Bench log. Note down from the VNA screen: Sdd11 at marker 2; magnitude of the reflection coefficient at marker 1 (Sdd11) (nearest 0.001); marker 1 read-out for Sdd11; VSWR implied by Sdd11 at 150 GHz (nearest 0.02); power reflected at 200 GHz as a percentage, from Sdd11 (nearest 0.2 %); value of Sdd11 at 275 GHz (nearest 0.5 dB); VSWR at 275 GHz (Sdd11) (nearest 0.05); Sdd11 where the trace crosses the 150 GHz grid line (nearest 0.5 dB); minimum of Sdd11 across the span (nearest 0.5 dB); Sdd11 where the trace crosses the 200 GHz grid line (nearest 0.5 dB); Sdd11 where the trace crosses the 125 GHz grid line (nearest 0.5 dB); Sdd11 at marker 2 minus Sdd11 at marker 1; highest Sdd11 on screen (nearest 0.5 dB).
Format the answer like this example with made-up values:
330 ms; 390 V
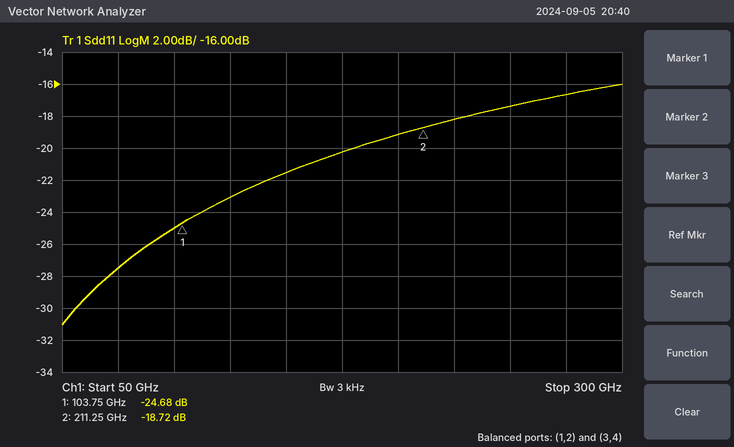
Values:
-18.72 dB; 0.058; -24.68 dB; 1.18; 1.2 %; -16.5 dB; 1.35; -21.5 dB; -31.0 dB; -19.0 dB; -23.0 dB; 5.96 dB; -16.0 dB
